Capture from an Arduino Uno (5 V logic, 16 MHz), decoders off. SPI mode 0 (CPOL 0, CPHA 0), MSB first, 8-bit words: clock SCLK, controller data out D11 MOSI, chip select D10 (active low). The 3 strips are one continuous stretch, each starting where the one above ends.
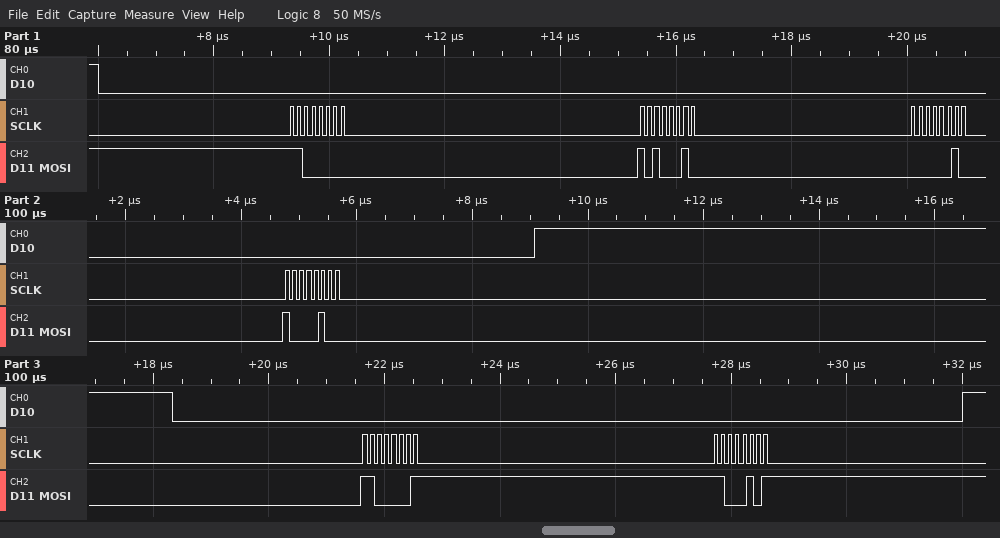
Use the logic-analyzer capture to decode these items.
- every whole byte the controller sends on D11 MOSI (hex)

C0 A2 02 84 C1 C5
